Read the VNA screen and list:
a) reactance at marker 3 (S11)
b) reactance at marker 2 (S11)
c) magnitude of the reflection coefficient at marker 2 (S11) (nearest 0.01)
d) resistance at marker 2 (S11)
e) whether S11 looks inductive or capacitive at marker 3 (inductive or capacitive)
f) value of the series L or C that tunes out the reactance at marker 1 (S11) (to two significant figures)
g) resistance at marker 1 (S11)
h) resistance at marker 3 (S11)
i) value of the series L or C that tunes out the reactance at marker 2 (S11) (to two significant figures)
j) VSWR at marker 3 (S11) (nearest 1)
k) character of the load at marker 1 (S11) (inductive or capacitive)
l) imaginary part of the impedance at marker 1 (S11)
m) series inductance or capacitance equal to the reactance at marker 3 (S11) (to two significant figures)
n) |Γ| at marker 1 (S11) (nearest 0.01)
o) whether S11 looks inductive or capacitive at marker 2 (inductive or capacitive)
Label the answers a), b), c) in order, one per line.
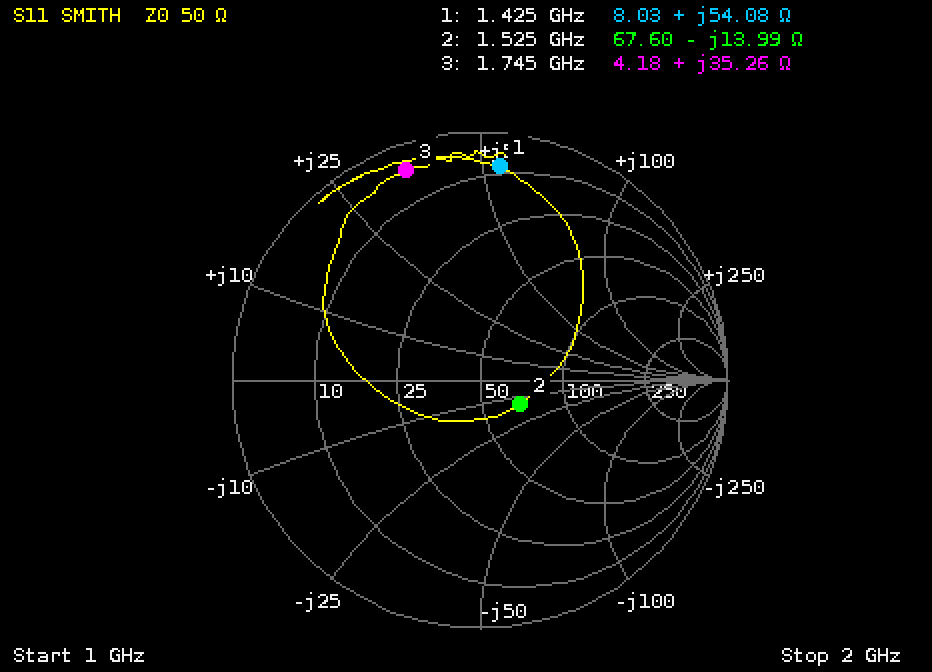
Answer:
a) +35.26 Ω
b) -13.99 Ω
c) 0.19
d) 67.60 Ω
e) inductive
f) 2.1 pF
g) 8.03 Ω
h) 4.18 Ω
i) 1.5 nH
j) 18
k) inductive
l) +54.08 Ω
m) 3.2 nH
n) 0.86
o) capacitive
